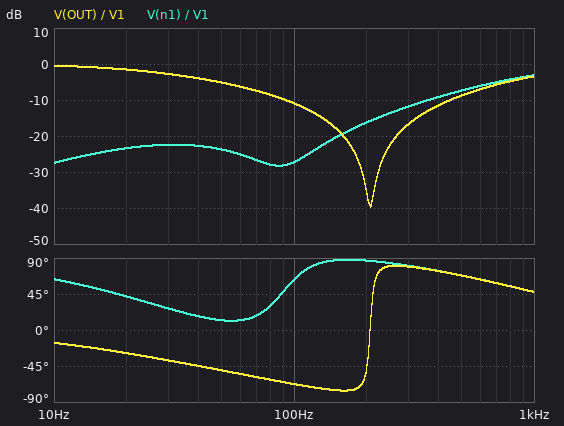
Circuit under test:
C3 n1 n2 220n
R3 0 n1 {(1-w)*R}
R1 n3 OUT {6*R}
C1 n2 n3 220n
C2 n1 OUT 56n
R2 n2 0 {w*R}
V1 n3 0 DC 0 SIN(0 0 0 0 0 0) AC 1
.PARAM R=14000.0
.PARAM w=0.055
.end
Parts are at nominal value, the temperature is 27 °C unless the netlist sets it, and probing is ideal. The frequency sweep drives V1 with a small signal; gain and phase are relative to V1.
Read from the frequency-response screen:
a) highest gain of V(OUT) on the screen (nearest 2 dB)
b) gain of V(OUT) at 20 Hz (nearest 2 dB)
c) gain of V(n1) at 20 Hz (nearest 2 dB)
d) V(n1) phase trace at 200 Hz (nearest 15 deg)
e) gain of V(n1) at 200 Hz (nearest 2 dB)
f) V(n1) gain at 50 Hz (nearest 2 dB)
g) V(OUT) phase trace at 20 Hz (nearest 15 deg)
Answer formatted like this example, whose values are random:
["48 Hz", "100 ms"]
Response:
["0 dB", "-2 dB", "-24 dB", "90 deg", "-16 dB", "-24 dB", "-30 deg"]
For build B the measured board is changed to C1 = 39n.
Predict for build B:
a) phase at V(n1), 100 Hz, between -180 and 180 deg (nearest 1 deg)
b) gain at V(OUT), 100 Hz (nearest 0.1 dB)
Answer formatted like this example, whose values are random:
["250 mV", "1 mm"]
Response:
["-28 deg", "-9.2 dB"]
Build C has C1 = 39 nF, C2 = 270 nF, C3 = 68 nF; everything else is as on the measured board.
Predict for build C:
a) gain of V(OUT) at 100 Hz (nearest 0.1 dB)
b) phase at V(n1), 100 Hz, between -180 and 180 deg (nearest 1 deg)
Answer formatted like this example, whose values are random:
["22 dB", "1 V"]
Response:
["-16.4 dB", "-22 deg"]
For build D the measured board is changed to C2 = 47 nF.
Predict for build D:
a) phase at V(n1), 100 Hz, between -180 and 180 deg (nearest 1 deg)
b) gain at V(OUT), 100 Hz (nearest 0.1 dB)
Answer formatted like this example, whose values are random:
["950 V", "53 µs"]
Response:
["64 deg", "-9.5 dB"]
